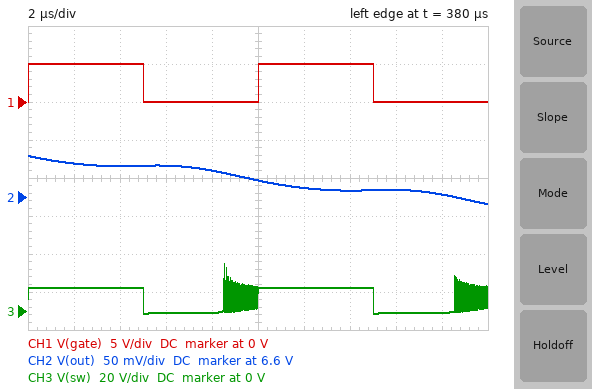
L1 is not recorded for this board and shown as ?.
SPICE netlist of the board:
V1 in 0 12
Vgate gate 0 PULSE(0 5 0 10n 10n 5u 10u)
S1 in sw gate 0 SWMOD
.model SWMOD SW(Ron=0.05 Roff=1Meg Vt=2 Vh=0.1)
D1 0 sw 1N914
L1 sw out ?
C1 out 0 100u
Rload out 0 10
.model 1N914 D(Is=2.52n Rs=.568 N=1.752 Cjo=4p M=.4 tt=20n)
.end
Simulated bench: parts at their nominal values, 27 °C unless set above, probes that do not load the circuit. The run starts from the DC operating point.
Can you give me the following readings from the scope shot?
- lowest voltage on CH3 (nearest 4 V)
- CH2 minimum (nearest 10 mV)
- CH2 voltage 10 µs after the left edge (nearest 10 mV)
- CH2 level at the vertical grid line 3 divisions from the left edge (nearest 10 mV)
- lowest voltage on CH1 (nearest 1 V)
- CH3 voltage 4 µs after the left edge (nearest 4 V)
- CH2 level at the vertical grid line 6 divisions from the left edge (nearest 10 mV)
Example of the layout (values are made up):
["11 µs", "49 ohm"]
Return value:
["0 V", "6.59 V", "6.62 V", "6.64 V", "0 V", "12 V", "6.61 V"]
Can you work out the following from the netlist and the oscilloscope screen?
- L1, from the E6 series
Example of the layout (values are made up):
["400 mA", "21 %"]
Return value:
["33 µH"]
